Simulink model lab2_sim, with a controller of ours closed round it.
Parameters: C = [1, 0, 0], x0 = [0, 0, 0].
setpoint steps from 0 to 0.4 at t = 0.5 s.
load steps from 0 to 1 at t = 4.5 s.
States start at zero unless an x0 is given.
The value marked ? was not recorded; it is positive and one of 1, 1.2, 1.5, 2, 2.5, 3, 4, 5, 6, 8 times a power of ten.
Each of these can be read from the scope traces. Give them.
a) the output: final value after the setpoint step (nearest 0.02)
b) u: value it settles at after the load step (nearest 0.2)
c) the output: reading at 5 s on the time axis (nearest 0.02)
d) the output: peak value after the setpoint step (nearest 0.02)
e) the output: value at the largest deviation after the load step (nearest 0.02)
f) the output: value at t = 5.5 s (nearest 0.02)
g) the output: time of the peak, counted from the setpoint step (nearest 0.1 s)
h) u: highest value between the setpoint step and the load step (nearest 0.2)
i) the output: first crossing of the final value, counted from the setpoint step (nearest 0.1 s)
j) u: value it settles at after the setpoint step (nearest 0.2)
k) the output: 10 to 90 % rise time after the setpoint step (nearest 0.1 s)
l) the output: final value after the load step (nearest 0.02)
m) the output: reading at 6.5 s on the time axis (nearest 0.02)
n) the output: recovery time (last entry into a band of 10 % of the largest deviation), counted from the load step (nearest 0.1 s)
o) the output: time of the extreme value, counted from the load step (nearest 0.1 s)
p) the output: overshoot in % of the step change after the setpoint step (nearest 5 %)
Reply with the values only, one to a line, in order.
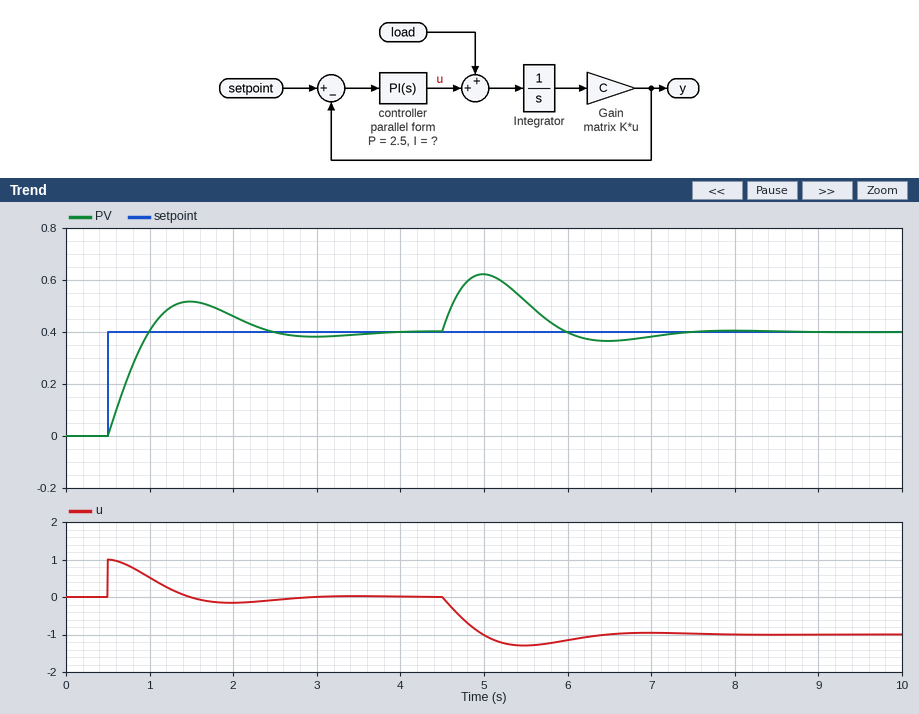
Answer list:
0.40
-1.0
0.62
0.52
0.62
0.52
1.0 s
1.0
0.5 s
0.0
0.4 s
0.40
0.36
2.4 s
0.5 s
30 %
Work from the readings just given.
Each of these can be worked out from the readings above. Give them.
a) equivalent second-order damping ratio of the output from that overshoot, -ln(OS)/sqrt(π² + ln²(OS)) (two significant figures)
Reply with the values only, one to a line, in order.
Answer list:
0.36
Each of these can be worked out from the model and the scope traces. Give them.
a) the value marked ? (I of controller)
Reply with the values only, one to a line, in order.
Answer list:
6
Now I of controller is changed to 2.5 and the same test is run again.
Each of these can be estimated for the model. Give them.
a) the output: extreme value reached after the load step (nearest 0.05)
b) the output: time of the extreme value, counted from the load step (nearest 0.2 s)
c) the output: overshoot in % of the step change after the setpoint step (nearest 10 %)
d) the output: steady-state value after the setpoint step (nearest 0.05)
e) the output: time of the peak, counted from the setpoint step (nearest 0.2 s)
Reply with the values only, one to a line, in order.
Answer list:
0.65
0.6 s
20 %
0.40
1.4 s
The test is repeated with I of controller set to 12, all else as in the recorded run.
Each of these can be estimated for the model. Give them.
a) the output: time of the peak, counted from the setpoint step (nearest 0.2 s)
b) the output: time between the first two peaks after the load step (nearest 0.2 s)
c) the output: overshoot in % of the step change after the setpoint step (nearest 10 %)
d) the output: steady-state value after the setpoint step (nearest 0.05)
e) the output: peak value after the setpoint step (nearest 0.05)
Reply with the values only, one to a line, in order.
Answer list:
0.8 s
2.0 s
40 %
0.40
0.55
